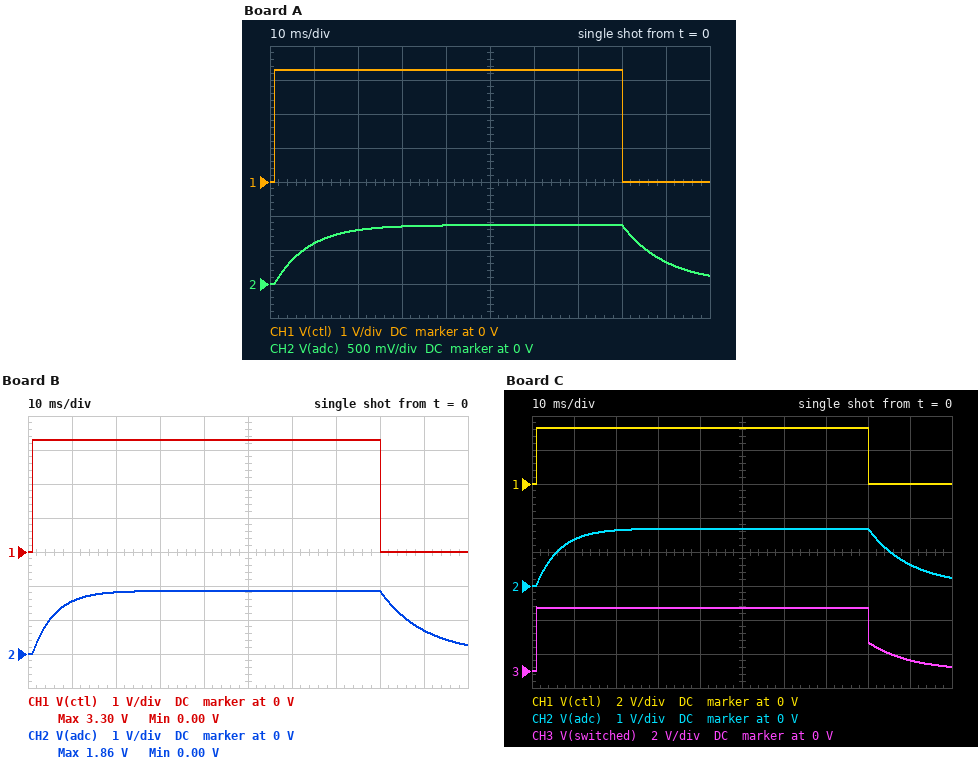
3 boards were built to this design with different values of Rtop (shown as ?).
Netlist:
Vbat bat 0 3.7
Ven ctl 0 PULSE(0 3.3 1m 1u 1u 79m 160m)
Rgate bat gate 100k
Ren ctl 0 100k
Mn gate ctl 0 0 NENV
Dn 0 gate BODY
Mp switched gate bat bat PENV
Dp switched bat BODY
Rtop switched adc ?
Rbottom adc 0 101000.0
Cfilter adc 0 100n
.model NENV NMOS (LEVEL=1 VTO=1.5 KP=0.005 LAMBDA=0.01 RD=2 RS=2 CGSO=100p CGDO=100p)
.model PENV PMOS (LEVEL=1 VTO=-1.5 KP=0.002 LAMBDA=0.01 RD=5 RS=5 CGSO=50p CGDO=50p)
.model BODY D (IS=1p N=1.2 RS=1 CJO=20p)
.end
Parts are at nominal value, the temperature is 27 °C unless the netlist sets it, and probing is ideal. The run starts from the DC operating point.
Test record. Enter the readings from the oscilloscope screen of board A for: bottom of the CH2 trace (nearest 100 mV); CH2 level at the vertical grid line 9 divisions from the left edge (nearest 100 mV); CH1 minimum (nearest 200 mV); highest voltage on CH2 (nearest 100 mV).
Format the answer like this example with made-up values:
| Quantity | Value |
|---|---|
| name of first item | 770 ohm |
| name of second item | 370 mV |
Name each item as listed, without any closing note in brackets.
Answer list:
| Quantity | Value |
|---|---|
| bottom of the CH2 trace | 0 V |
| CH2 level at the vertical grid line 9 divisions from the left edge | 300 mV |
| CH1 minimum | 0 V |
| highest voltage on CH2 | 900 mV |
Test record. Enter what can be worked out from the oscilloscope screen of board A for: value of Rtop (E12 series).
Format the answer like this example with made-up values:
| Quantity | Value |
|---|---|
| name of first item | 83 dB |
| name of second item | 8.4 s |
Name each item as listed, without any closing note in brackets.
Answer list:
| Quantity | Value |
|---|---|
| value of Rtop | 330 kΩ |
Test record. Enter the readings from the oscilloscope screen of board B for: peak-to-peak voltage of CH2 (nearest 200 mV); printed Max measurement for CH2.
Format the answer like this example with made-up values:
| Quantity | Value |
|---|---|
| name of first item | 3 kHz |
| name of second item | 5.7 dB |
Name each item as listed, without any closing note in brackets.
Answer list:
| Quantity | Value |
|---|---|
| peak-to-peak voltage of CH2 | 1.8 V |
| printed Max measurement for CH2 | 1.86 V |
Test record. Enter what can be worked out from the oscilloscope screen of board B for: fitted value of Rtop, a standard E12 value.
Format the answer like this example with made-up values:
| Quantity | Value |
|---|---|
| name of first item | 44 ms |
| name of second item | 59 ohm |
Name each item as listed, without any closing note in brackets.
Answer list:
| Quantity | Value |
|---|---|
| fitted value of Rtop, a standard E12 value | 100 kΩ |
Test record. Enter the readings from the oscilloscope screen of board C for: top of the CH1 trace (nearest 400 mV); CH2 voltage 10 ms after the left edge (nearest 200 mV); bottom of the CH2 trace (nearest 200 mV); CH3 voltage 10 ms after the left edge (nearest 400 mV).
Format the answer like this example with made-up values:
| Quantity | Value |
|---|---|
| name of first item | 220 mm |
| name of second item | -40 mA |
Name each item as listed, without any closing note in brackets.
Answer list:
| Quantity | Value |
|---|---|
| top of the CH1 trace | 3.2 V |
| CH2 voltage 10 ms after the left edge | 1.4 V |
| bottom of the CH2 trace | 0 V |
| CH3 voltage 10 ms after the left edge | 3.6 V |
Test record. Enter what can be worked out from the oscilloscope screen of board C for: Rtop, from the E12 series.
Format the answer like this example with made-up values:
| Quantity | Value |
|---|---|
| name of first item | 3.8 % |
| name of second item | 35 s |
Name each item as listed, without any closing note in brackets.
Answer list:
| Quantity | Value |
|---|---|
| Rtop, from the E12 series | 120 kΩ |
